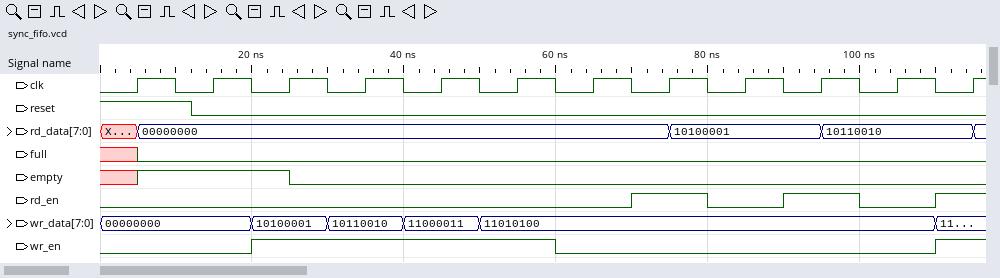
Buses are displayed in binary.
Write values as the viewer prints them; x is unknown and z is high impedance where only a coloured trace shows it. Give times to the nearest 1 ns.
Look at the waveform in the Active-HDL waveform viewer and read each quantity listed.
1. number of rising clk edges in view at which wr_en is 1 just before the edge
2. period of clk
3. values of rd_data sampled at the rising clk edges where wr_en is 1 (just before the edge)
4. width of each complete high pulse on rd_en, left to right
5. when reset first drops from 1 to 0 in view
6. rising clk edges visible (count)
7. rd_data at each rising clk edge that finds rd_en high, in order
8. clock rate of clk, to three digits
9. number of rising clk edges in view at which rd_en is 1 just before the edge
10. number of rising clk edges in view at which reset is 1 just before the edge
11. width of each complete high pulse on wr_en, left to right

5
10 ns
00000000, 00000000, 00000000, 00000000, 10110010
10 ns, 10 ns
12 ns
12
00000000, 10100001, 10110010
100 MHz
3
1
40 ns
